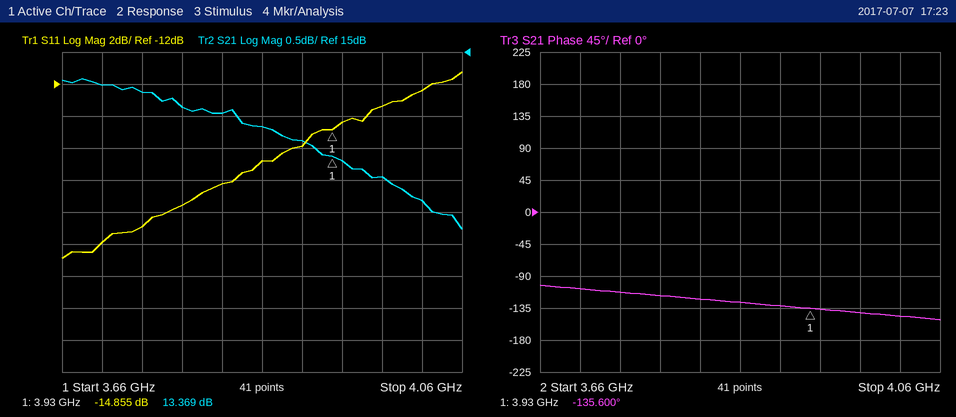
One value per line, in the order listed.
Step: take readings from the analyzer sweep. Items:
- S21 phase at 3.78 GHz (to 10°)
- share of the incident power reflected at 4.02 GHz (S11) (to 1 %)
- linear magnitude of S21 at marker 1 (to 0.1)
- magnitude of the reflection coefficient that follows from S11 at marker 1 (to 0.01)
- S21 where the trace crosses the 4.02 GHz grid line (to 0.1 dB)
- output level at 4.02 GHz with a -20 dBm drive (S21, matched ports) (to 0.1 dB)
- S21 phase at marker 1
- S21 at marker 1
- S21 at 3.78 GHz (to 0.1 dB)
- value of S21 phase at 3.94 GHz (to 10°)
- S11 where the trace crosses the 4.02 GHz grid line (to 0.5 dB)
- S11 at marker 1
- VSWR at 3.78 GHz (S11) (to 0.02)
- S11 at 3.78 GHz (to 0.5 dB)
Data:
-120°
6 %
4.7
0.18
12.7 dB
-7.3 dBm
-135.600°
13.369 dB
14.1 dB
-140°
-12.5 dB
-14.855 dB
1.24
-19.5 dB
